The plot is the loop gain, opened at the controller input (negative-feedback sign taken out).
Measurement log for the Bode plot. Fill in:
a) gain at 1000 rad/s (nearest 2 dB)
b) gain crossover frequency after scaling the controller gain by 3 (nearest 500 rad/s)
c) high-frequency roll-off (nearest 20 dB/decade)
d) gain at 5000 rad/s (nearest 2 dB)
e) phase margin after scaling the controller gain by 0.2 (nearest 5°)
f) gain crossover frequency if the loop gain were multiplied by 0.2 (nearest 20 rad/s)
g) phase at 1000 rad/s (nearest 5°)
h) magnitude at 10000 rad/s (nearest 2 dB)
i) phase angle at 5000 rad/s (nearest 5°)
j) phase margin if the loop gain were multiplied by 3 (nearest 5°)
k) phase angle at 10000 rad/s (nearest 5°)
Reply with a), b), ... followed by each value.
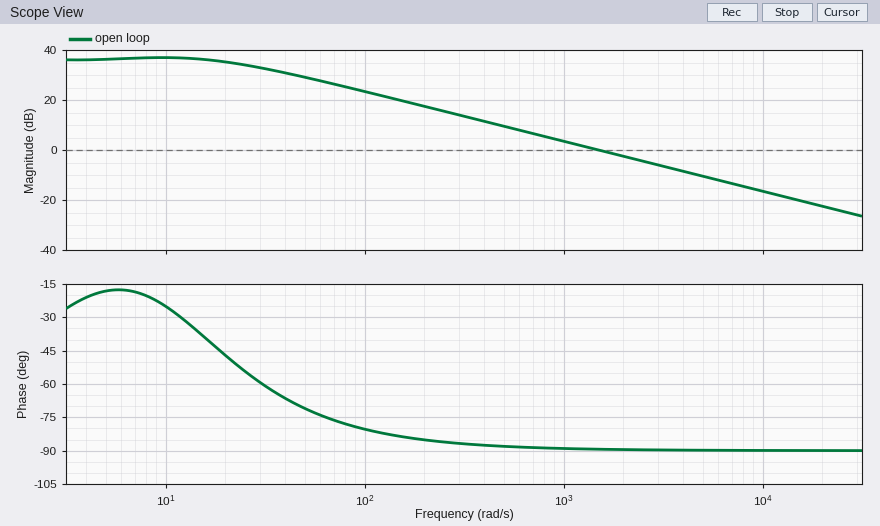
a) 4 dB
b) 4500 rad/s
c) -20 dB/decade
d) -10 dB
e) 95°
f) 300 rad/s
g) -90°
h) -16 dB
i) -90°
j) 90°
k) -90°
